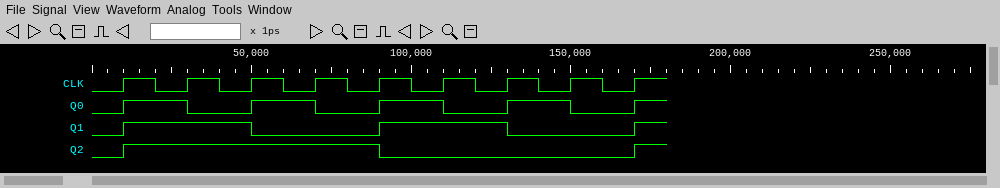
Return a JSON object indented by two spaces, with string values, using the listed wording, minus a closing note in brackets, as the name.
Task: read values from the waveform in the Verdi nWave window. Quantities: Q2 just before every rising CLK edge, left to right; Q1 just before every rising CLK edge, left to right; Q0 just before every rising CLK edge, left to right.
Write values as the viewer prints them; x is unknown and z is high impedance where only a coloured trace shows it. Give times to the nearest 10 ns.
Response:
{
  "Q2 just before every rising CLK edge, left to right": "0 1 1 1 1 0 0 0 0",
  "Q1 just before every rising CLK edge, left to right": "0 1 1 0 0 1 1 0 0",
  "Q0 just before every rising CLK edge, left to right": "0 1 0 1 0 1 0 1 0"
}
